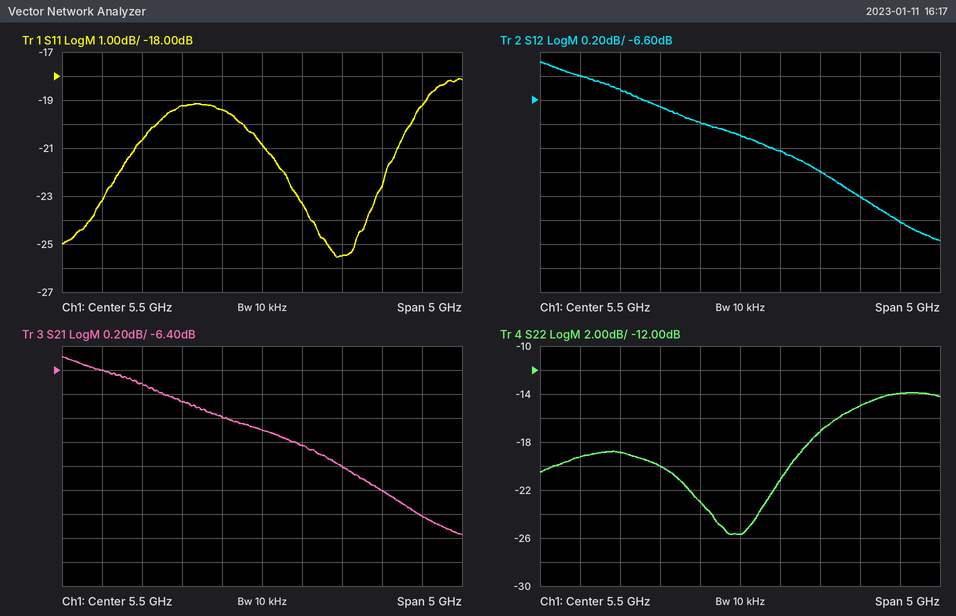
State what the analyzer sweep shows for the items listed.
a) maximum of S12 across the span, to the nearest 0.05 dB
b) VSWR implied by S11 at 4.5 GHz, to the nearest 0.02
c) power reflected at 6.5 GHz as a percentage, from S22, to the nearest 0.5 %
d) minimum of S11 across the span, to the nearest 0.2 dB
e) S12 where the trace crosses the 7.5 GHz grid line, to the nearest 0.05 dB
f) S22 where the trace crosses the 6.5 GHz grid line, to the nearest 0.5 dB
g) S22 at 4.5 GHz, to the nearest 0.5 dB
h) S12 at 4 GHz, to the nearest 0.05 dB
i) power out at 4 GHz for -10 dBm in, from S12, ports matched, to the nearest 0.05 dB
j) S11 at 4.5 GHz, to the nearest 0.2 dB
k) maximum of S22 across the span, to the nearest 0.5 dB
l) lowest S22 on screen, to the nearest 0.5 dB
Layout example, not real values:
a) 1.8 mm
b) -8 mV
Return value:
a) -6.30 dB
b) 1.24
c) 2.0 %
d) -25.6 dB
e) -7.60 dB
f) -17.0 dB
g) -20.0 dB
h) -6.50 dB
i) -16.50 dBm
j) -19.2 dB
k) -14.0 dB
l) -25.5 dB
